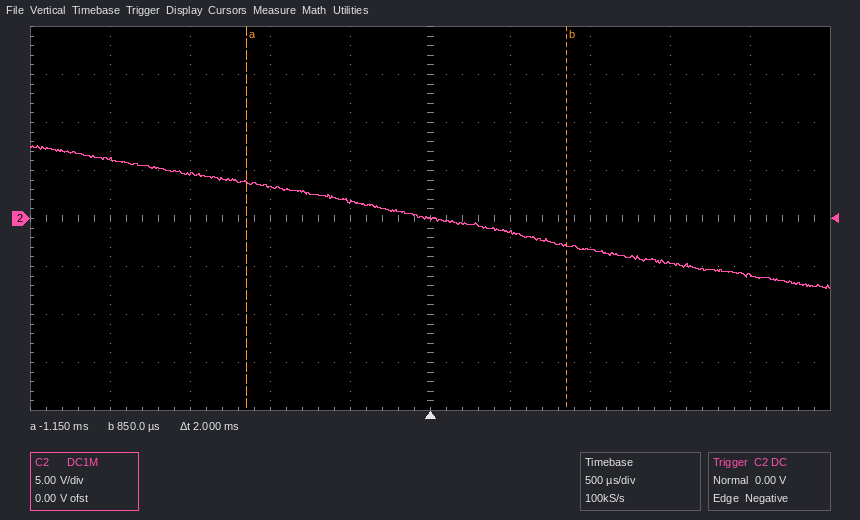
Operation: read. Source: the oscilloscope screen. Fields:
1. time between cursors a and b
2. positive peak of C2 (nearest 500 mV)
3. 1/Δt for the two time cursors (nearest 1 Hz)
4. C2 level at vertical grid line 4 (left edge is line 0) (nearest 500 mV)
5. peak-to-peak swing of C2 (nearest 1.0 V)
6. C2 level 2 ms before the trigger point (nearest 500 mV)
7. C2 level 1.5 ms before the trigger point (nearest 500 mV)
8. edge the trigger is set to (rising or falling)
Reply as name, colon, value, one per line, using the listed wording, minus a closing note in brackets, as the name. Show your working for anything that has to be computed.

time between cursors a and b: 2 ms
positive peak of C2: 7.5 V
1/Δt for the two time cursors: 1 / 2 ms ≈ 500 Hz
C2 level at vertical grid line 4 (left edge is line 0): 2.0 V
peak-to-peak swing of C2: 15.0 V
C2 level 2 ms before the trigger point: 6.0 V
C2 level 1.5 ms before the trigger point: 4.5 V
edge the trigger is set to: falling
